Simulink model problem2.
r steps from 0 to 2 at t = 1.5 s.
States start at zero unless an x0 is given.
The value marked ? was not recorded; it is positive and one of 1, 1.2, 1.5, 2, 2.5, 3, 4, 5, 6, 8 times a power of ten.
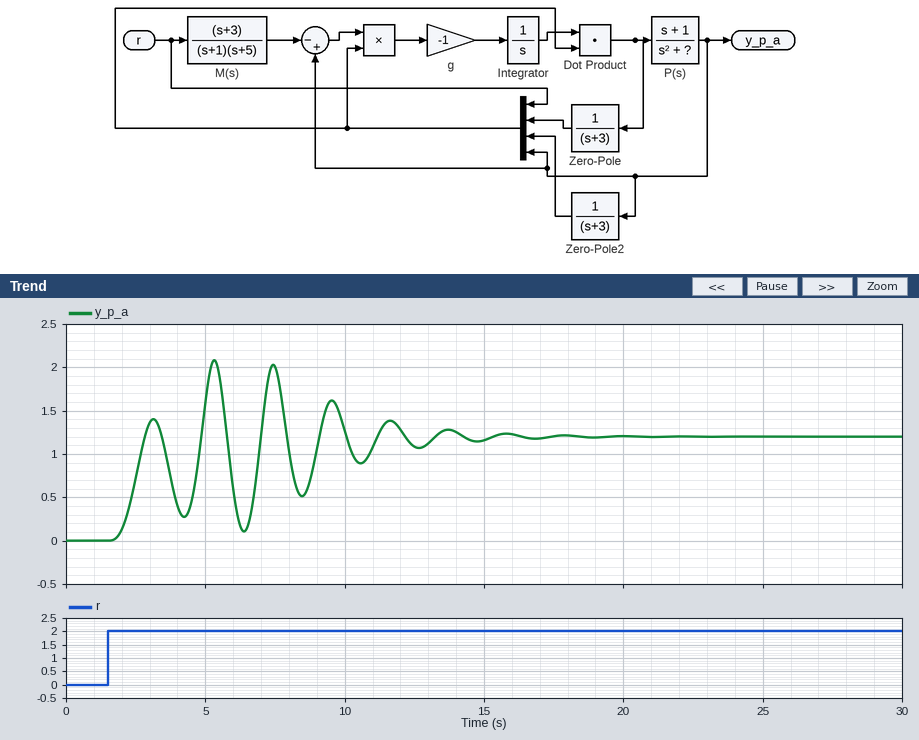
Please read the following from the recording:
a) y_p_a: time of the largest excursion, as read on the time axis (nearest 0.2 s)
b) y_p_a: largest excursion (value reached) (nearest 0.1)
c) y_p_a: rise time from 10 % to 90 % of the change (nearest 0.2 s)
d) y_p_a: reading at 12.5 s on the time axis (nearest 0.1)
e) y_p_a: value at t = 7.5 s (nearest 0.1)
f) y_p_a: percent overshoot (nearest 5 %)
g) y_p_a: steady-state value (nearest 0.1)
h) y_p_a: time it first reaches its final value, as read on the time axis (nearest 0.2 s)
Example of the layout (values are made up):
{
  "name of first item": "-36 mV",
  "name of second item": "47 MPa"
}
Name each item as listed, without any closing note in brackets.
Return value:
{
  "y_p_a: time of the largest excursion, as read on the time axis": "5.4 s",
  "y_p_a: largest excursion (value reached)": "2.1",
  "y_p_a: rise time from 10 % to 90 % of the change": "0.8 s",
  "y_p_a: reading at 12.5 s on the time axis": "1.1",
  "y_p_a: value at t = 7.5 s": "2.0",
  "y_p_a: percent overshoot": "75 %",
  "y_p_a: steady-state value": "1.2",
  "y_p_a: time it first reaches its final value, as read on the time axis": "2.8 s"
}
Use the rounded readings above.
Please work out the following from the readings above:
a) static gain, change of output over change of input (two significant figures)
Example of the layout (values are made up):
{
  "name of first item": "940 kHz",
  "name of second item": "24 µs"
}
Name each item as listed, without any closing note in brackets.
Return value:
{
  "static gain, change of output over change of input": "0.60"
}
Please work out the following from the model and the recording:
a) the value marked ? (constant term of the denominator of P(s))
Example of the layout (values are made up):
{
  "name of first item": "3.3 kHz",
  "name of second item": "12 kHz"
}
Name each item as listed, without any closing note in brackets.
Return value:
{
  "the value marked ? (constant term of the denominator of P(s))": "2"
}
